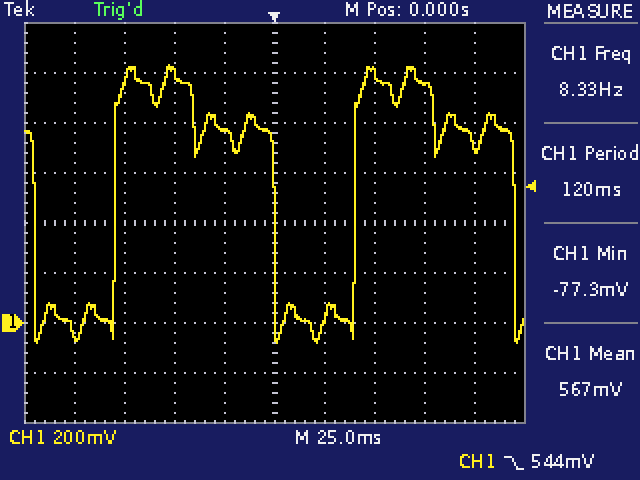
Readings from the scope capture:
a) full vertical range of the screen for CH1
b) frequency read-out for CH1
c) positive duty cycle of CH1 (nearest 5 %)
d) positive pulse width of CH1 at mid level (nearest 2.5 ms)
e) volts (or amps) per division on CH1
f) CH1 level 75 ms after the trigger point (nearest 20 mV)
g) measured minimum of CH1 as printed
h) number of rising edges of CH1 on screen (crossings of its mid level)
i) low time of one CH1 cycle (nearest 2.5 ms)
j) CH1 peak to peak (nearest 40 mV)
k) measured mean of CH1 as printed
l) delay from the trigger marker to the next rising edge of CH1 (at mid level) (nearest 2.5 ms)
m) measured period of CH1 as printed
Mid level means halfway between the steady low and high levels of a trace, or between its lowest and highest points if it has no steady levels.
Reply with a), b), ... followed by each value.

a) 1.6 V
b) 8.33 Hz
c) 65 %
d) 80.0 ms
e) 200 mV
f) 960 mV
g) -77.3 mV
h) 2
i) 40.0 ms
j) 1.12 V
k) 567 mV
l) 40.0 ms
m) 120 ms
